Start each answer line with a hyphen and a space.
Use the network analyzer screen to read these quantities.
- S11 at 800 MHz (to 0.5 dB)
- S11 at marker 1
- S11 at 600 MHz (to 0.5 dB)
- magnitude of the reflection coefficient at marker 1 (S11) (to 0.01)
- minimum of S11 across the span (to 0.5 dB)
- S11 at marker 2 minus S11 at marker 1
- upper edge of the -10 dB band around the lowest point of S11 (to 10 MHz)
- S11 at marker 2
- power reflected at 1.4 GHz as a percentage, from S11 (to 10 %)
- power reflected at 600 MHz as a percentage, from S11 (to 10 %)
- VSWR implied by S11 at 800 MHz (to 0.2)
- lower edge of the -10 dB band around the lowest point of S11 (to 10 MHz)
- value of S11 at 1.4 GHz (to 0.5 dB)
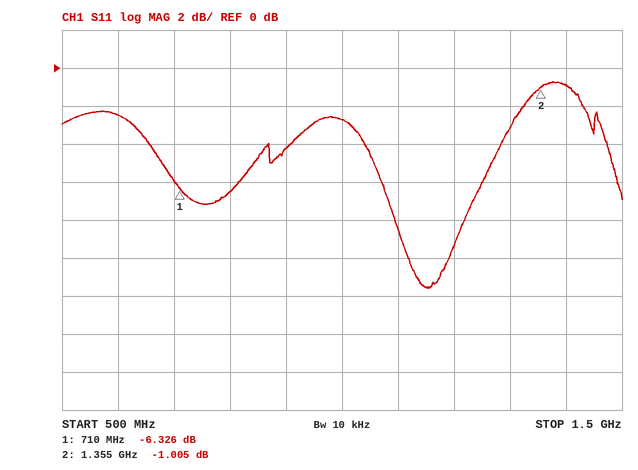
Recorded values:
- -6.5 dB
- -6.326 dB
- -2.5 dB
- 0.48
- -11.5 dB
- 5.321 dB
- 1.19 GHz
- -1.005 dB
- 80 %
- 60 %
- 2.8
- 1.12 GHz
- -1.0 dB
